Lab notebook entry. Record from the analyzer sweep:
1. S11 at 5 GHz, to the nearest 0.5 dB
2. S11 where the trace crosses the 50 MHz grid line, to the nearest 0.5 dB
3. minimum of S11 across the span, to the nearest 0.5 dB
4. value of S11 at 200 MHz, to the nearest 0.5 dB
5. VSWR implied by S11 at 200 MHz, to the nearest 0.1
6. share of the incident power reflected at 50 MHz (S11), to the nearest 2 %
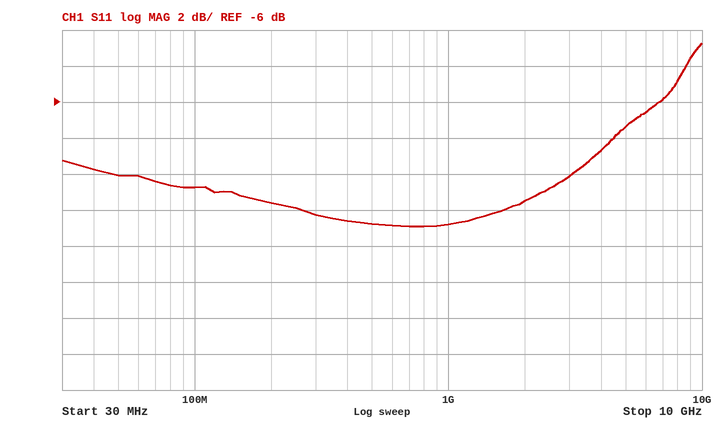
-7.5 dB
-10.0 dB
-13.0 dB
-11.5 dB
1.7
10 %
